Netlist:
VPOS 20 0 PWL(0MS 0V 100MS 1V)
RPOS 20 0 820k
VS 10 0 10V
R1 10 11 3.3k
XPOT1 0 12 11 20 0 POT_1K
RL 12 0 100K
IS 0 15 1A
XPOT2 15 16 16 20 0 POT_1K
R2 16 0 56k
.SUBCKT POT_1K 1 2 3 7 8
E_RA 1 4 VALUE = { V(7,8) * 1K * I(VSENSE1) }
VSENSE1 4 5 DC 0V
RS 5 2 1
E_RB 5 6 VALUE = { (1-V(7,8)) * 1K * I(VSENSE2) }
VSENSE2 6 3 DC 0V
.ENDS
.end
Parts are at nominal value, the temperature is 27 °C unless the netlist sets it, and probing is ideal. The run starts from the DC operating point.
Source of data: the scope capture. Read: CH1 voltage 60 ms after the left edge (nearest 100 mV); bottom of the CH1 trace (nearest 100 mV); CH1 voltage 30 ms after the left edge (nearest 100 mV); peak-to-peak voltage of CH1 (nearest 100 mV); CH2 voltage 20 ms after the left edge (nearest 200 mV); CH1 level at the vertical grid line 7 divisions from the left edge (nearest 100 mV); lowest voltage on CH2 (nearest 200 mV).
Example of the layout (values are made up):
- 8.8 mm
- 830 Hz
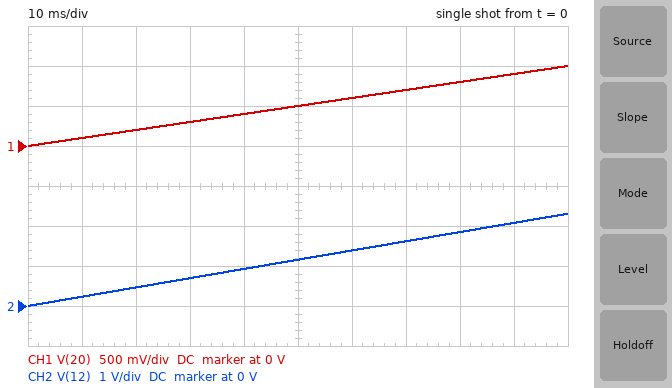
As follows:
- 600 mV
- 0 V
- 300 mV
- 1.0 V
- 400 mV
- 700 mV
- 0 V
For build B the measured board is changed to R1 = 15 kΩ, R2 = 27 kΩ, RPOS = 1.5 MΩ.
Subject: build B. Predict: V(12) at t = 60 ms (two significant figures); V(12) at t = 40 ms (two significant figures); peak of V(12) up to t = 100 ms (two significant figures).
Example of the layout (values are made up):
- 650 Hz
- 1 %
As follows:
- 370 mV
- 250 mV
- 620 mV
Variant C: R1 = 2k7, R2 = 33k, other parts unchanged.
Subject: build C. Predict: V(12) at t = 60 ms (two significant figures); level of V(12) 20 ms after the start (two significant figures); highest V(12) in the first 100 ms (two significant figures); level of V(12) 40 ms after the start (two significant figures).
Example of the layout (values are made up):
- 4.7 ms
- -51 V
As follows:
- 1.6 V
- 540 mV
- 2.7 V
- 1.1 V
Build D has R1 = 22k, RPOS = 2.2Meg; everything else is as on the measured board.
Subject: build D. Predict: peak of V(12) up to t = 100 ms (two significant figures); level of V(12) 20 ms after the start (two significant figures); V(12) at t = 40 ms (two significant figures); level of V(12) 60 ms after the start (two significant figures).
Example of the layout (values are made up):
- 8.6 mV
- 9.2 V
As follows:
- 430 mV
- 87 mV
- 170 mV
- 260 mV
